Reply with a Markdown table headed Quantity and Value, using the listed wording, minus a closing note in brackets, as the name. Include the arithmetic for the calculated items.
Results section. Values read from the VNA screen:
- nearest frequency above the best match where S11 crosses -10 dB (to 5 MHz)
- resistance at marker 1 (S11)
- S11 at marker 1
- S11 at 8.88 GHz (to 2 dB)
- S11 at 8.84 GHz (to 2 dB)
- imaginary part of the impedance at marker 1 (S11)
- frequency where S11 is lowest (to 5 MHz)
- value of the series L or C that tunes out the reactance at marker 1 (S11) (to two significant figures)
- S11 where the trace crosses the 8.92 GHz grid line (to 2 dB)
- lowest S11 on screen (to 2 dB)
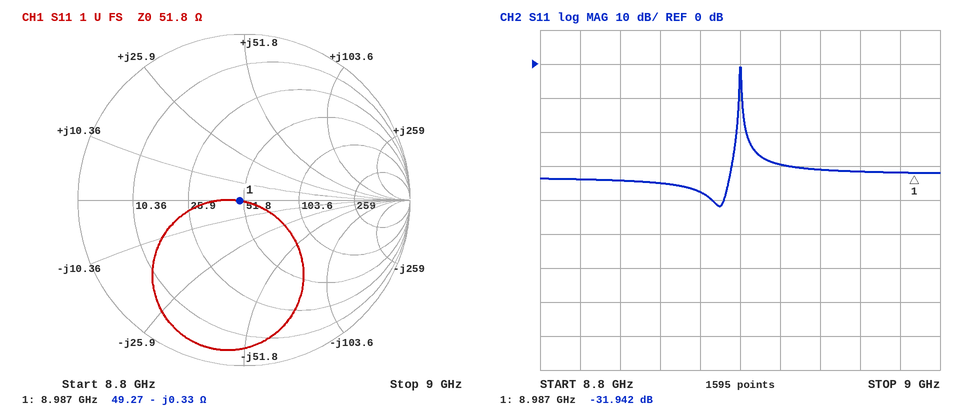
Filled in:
| Quantity | Value |
|---|---|
| nearest frequency above the best match where S11 crosses -10 dB | 8.900 GHz |
| resistance at marker 1 | 49.27 Ω |
| S11 at marker 1 | -31.942 dB |
| S11 at 8.88 GHz | -38 dB |
| S11 at 8.84 GHz | -34 dB |
| imaginary part of the impedance at marker 1 | -0.33 Ω |
| frequency where S11 is lowest | 8.890 GHz |
| value of the series L or C that tunes out the reactance at marker 1 (S11) | L = 0.33 Ω/(2π × 8.987 GHz) ≈ 5.8 pH |
| S11 where the trace crosses the 8.92 GHz grid line | -30 dB |
| lowest S11 on screen | -42 dB |
